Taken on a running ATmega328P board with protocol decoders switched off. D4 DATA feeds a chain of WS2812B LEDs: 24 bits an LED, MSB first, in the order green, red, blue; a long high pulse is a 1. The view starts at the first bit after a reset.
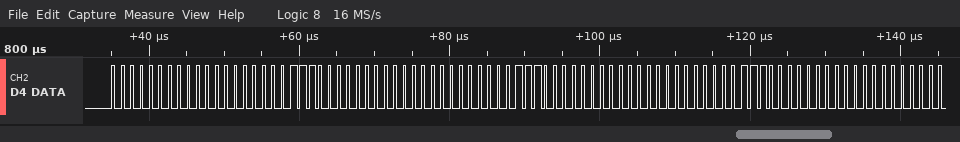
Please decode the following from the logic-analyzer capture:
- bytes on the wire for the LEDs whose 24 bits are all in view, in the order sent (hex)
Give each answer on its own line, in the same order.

00 00 1C 00 00 1C 00 00 1C
